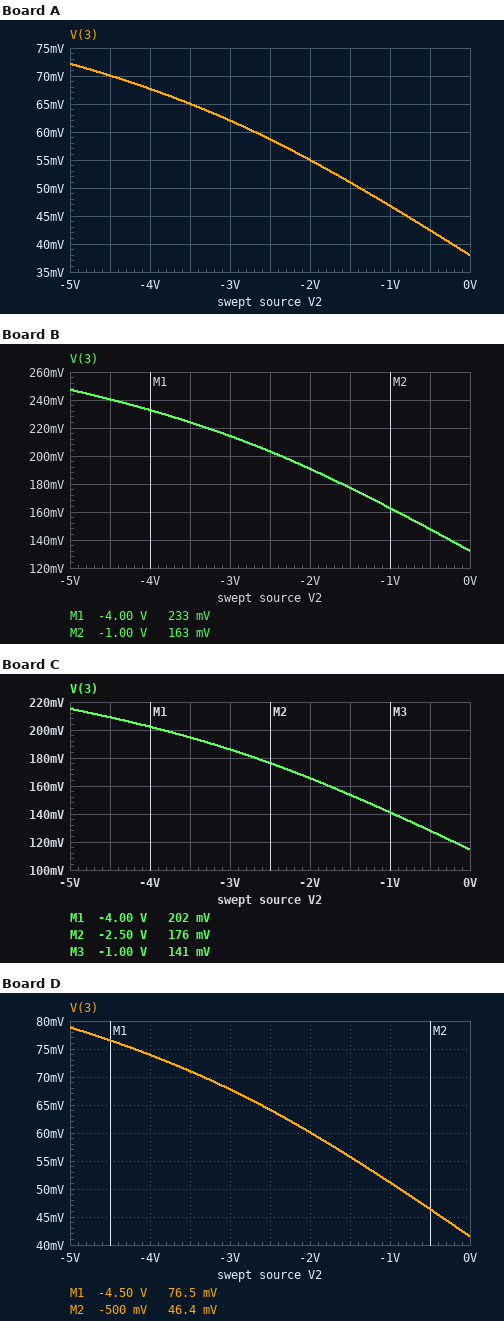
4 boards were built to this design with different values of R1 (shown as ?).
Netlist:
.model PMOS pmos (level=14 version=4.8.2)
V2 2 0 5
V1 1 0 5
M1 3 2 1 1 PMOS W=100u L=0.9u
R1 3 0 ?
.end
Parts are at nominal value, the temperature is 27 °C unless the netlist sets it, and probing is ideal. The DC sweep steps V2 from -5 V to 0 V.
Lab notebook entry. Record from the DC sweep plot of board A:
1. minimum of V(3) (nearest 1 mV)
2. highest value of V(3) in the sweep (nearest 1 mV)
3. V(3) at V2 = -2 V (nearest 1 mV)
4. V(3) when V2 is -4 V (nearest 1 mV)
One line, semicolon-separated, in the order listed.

38 mV; 72 mV; 55 mV; 68 mV
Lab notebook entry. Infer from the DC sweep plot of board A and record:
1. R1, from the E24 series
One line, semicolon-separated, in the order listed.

0.43 Ω
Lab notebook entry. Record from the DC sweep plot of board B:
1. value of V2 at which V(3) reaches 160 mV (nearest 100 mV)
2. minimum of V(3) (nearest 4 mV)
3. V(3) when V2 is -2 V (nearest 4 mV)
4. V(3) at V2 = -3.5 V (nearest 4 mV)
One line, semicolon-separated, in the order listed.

-900 mV; 132 mV; 192 mV; 224 mV
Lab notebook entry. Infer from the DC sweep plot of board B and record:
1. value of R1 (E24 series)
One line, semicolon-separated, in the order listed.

1.5 Ω
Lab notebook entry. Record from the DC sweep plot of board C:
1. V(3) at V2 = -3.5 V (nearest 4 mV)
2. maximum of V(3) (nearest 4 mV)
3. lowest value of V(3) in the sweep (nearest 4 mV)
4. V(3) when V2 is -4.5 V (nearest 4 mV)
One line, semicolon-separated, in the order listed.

196 mV; 216 mV; 116 mV; 208 mV
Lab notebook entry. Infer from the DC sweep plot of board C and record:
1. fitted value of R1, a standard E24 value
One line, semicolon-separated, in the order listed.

1.3 Ω
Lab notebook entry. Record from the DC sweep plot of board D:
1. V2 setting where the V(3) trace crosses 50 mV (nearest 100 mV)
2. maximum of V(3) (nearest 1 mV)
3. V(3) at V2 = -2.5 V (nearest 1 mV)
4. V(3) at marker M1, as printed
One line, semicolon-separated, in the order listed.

-900 mV; 79 mV; 64 mV; 76.5 mV
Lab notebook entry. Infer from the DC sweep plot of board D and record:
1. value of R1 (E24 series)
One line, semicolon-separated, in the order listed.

0.47 Ω
